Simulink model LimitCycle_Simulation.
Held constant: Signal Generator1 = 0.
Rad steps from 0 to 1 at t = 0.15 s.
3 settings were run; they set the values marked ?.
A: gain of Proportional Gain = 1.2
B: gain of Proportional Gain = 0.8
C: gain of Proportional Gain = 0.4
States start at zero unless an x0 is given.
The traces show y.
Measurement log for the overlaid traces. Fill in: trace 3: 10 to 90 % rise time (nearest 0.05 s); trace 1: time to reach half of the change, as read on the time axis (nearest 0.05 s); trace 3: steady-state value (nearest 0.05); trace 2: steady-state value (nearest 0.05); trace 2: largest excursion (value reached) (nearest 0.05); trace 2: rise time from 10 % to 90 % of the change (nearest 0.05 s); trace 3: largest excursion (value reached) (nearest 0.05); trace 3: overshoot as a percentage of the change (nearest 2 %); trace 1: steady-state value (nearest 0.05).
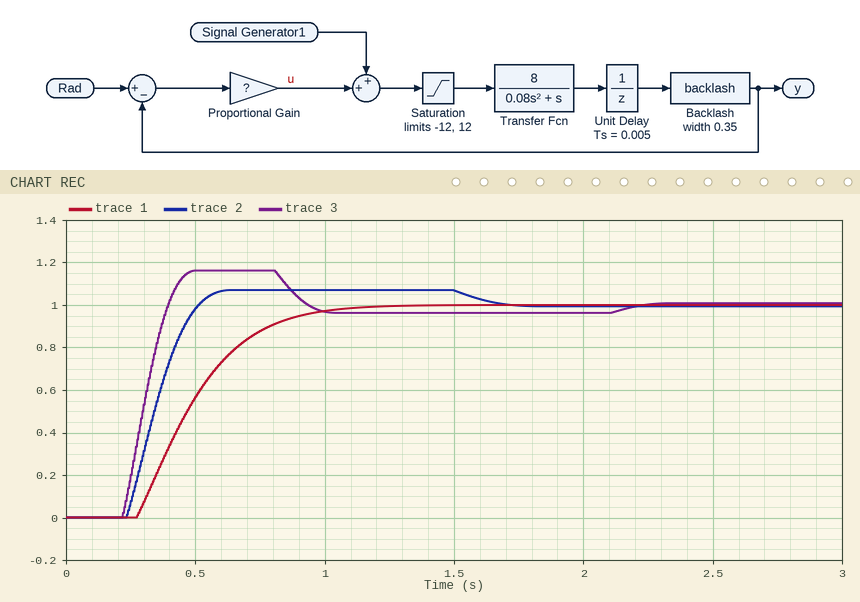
0.15 s
0.45 s
1.00
1.00
1.05
0.20 s
1.15
16 %
1.00
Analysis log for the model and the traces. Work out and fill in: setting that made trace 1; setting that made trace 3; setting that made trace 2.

C
A
B
